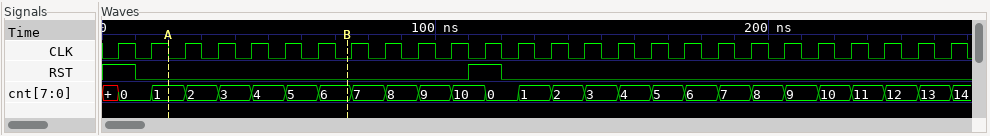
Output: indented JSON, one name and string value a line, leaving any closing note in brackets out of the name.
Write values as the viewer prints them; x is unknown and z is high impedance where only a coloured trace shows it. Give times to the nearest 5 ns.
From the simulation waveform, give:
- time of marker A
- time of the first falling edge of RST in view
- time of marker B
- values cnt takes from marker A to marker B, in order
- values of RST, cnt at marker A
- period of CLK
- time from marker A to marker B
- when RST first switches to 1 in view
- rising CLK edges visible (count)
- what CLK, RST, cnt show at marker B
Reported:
{
  "time of marker A": "20 ns",
  "time of the first falling edge of RST in view": "10 ns",
  "time of marker B": "75 ns",
  "values cnt takes from marker A to marker B, in order": "1, 2, 3, 4, 5, 6",
  "values of RST, cnt at marker A": "RST=0, cnt=1",
  "period of CLK": "10 ns",
  "time from marker A to marker B": "55 ns",
  "when RST first switches to 1 in view": "110 ns",
  "rising CLK edges visible": "26",
  "what CLK, RST, cnt show at marker B": "CLK=0, RST=0, cnt=6"
}
